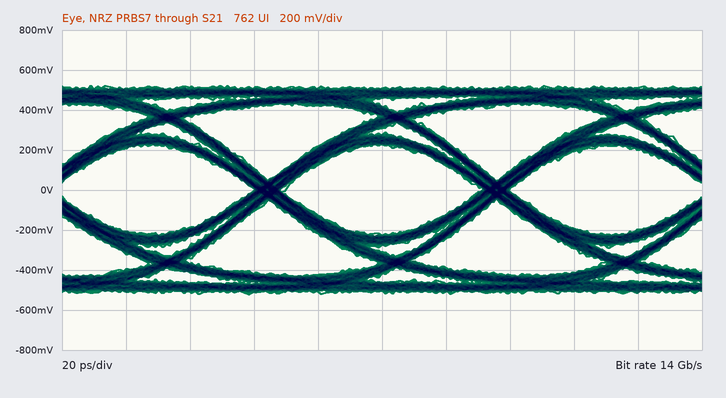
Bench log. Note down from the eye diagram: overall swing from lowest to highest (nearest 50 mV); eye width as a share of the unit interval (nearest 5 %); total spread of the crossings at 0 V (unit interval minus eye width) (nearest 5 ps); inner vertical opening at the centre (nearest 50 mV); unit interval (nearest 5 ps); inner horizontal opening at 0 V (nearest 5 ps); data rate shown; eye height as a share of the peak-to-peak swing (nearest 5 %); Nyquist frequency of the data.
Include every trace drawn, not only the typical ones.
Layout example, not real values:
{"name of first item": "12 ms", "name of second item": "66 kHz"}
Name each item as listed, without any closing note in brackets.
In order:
{"overall swing from lowest to highest": "1.05 V", "eye width as a share of the unit interval": "85 %", "total spread of the crossings at 0 V (unit interval minus eye width)": "10 ps", "inner vertical opening at the centre": "450 mV", "unit interval": "70 ps", "inner horizontal opening at 0 V": "60 ps", "data rate shown": "14 Gb/s", "eye height as a share of the peak-to-peak swing": "45 %", "Nyquist frequency of the data": "7 GHz"}
